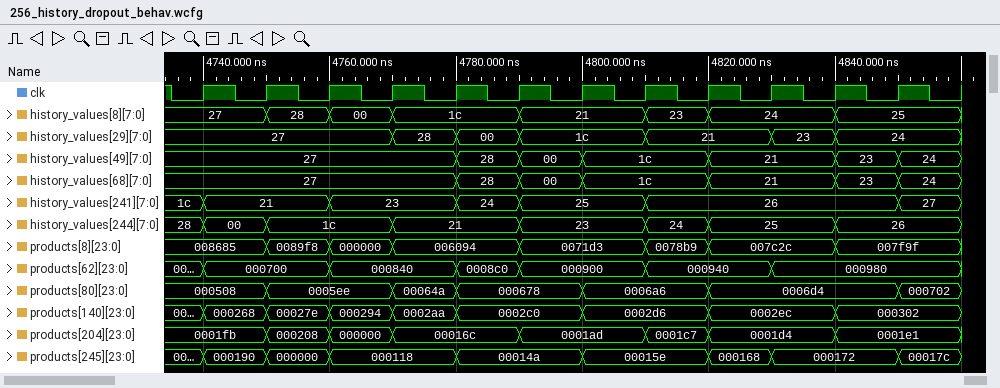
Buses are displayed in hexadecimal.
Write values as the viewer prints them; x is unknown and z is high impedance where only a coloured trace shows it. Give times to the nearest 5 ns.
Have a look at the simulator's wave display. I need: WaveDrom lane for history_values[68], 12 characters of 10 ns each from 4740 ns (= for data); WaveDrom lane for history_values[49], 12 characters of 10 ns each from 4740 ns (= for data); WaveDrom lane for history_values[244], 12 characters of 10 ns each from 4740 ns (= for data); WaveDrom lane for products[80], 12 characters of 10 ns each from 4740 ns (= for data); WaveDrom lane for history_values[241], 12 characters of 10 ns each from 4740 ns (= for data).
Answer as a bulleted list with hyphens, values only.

- {name: 'history_values[68]', wave: '=...===.=.==', data: '27 28 00 1c 21 23 24'}
- {name: 'history_values[49]', wave: '=...===.=.==', data: '27 28 00 1c 21 23 24'}
- {name: 'history_values[244]', wave: '==.=.=.==.=.', data: '00 1c 21 23 24 25 26'}
- {name: 'products[80]', wave: '==.==.=.=..=', data: '000508 0005ee 00064a 000678 0006a6 0006d4 000702'}
- {name: 'history_values[241]', wave: '=.=.==.=...=', data: '21 23 24 25 26 27'}
